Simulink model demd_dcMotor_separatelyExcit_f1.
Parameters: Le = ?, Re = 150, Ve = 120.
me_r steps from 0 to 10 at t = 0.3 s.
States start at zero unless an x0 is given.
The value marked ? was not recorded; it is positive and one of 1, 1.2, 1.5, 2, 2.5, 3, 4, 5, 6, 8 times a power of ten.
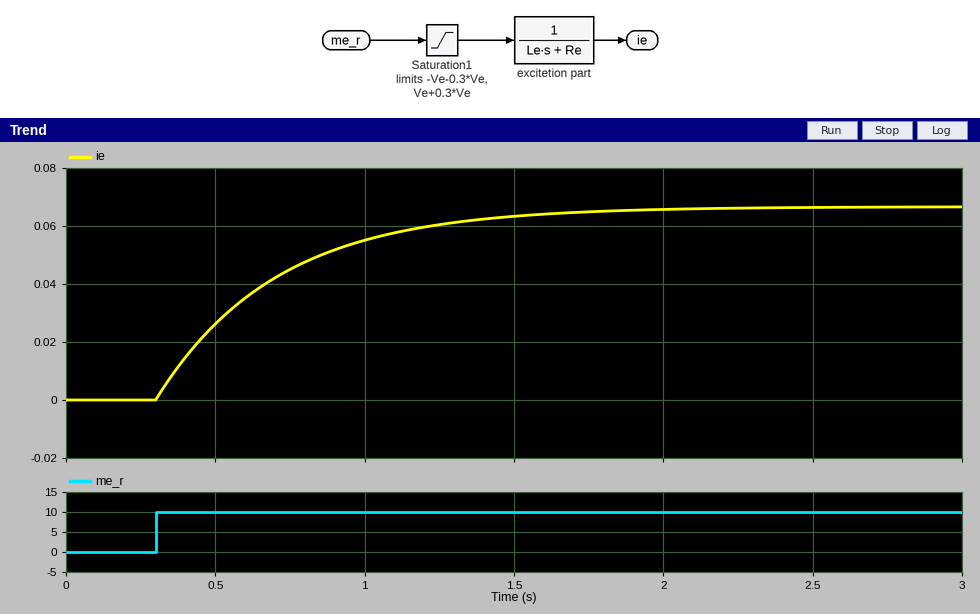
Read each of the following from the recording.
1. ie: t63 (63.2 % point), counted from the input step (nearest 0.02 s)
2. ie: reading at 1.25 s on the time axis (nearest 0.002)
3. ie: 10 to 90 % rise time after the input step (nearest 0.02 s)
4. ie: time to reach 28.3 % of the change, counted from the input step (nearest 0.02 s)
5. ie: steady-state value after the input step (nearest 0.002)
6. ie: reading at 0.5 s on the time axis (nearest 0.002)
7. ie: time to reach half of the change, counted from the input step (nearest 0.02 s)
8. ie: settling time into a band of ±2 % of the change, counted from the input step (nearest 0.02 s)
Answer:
0.40 s
0.060
0.88 s
0.14 s
0.066
0.026
0.28 s
1.56 s
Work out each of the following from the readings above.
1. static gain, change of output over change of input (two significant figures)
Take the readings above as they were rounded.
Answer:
0.0066
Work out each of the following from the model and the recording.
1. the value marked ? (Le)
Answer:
60
